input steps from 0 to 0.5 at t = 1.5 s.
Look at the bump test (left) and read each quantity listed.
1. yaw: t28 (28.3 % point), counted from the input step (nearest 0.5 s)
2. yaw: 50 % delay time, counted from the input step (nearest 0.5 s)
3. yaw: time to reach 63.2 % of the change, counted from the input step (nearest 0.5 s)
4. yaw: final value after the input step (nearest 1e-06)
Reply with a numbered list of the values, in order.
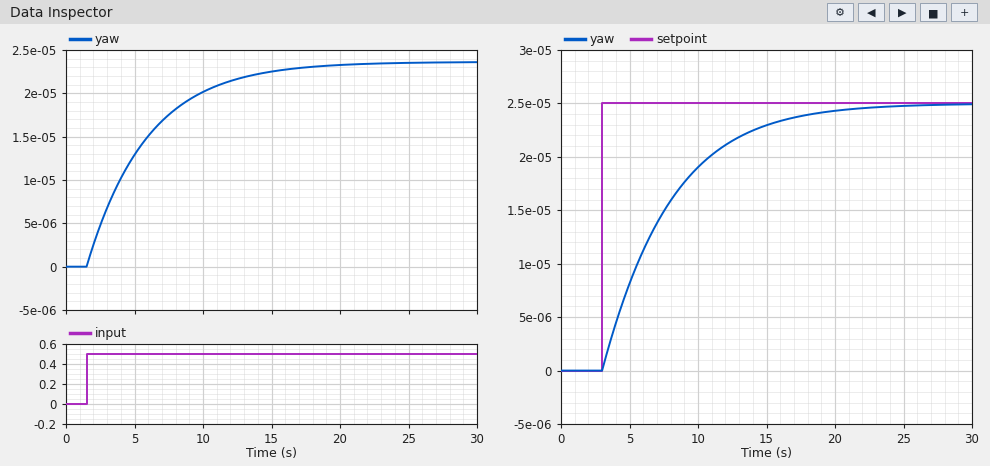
1. 1.5 s
2. 3.0 s
3. 4.5 s
4. 0.000024
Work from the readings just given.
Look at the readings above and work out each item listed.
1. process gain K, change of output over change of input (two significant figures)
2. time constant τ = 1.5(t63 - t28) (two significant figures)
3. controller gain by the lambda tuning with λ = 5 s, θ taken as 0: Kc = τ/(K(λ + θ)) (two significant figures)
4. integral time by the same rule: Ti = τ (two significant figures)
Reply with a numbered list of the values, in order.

1. 0.000048
2. 4.5 s
3. 19000
4. 4.5 s
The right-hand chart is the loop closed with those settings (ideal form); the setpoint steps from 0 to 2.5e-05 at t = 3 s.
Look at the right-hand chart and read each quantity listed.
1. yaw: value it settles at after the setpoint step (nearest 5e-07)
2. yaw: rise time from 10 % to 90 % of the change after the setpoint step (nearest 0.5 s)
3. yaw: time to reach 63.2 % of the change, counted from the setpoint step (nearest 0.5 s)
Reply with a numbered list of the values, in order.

1. 0.0000250
2. 10.5 s
3. 5.0 s
